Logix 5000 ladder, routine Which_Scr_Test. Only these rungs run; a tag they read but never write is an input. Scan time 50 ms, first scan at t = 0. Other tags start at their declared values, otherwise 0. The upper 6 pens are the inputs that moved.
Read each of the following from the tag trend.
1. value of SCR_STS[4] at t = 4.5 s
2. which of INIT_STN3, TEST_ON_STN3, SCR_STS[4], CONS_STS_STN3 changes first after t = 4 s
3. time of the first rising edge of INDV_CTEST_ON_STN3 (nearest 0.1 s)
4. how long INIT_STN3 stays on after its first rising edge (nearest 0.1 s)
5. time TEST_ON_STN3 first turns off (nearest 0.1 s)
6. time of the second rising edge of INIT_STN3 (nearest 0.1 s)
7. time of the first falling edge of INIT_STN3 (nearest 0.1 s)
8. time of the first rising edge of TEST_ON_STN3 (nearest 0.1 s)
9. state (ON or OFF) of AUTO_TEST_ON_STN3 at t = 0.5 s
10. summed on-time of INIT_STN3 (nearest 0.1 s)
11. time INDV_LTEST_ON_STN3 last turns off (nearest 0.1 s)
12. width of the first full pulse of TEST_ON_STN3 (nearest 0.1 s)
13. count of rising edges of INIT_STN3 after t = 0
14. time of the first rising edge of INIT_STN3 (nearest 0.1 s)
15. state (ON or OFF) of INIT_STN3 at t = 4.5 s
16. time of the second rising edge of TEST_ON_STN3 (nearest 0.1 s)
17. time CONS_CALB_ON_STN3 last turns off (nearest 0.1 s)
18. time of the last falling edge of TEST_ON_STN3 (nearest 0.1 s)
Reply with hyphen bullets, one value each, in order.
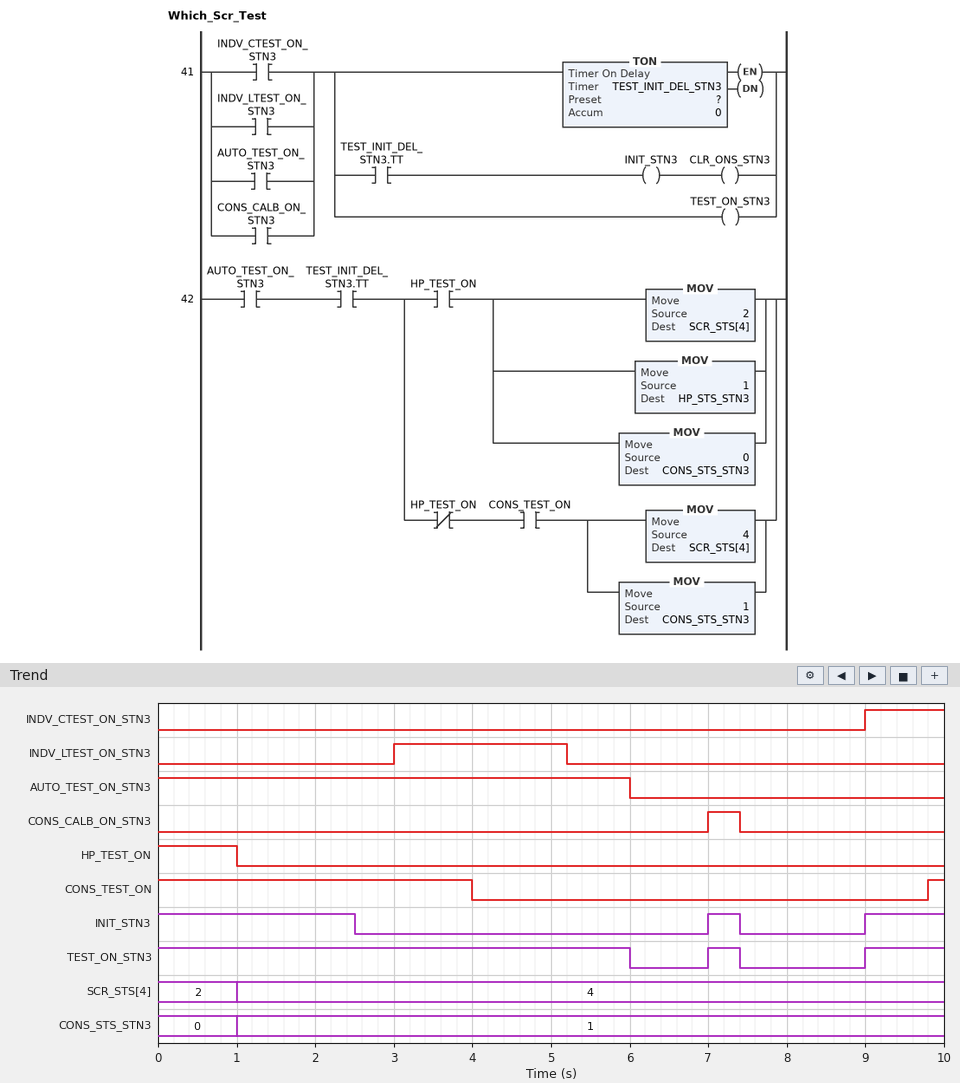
- 4
- TEST_ON_STN3
- 9.0 s
- 0.4 s
- 6.0 s
- 9.0 s
- 2.5 s
- 7.0 s
- ON
- 3.9 s
- 5.2 s
- 0.4 s
- 2
- 7.0 s
- OFF
- 9.0 s
- 7.4 s
- 7.4 s
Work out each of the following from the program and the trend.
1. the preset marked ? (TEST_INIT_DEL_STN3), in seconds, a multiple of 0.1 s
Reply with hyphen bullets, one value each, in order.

- 2.5 s
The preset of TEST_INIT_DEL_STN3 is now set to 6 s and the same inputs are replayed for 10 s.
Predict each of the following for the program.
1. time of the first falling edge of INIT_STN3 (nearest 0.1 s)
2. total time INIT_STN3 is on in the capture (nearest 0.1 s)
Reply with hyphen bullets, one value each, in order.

- 6.0 s
- 7.4 s
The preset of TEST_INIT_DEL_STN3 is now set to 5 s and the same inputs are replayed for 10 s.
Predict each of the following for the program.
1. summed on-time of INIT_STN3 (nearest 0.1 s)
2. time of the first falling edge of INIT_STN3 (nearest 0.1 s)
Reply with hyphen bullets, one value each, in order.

- 6.4 s
- 5.0 s
